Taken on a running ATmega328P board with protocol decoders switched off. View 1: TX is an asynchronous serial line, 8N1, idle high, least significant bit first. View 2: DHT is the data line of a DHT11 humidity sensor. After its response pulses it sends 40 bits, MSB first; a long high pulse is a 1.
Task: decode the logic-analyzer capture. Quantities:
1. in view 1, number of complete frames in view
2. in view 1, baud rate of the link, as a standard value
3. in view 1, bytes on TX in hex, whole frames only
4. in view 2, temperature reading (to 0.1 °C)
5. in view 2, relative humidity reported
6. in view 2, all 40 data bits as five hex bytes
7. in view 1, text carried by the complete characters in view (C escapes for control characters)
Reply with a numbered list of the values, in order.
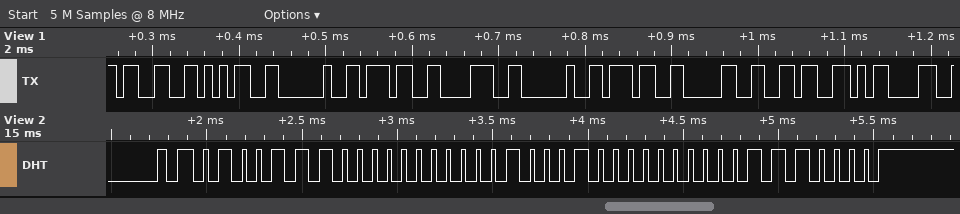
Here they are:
1. 10
2. 115200 baud
3. 33 35 20 37 38 20 37 30 36 0D
4. 34.0 °C
5. 78 %
6. 4E 00 22 00 70
7. "35 78 706\r"
